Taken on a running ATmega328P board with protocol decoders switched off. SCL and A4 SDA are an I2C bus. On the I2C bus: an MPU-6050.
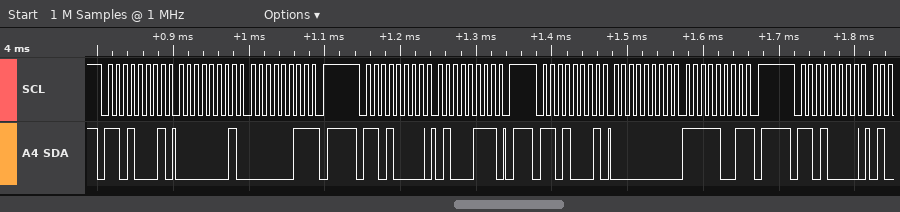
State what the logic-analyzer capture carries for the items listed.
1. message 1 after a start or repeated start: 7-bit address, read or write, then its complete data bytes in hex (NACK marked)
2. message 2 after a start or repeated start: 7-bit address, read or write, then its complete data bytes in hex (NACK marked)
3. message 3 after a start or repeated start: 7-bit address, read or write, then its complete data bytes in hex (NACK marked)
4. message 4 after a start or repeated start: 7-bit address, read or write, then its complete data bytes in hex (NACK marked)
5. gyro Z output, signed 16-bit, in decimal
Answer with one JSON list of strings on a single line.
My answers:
["0x68 read: 01 03 NACK", "0x68 write: 47", "0x68 read: 00 F9 NACK", "0x68 write", "249"]
